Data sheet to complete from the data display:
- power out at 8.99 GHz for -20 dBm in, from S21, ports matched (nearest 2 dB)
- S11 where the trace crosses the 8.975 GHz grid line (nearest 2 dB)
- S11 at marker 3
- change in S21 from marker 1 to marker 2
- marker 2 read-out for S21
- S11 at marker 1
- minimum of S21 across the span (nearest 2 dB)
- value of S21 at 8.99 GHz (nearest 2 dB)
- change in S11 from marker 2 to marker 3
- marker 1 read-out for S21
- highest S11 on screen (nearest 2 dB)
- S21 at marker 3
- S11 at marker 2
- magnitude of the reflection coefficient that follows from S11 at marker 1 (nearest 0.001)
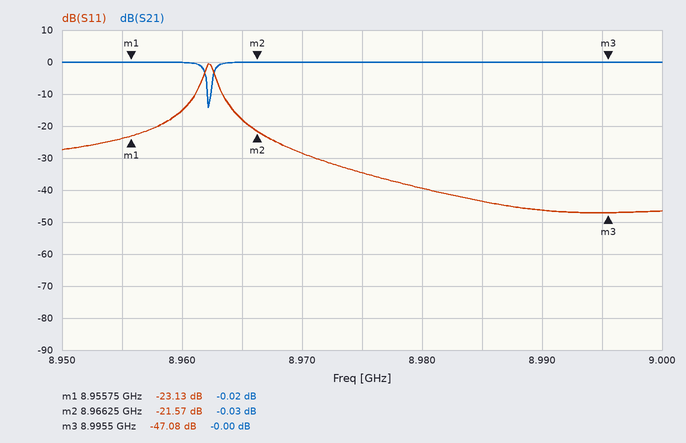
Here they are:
-20 dBm
-34 dB
-47.08 dB
-0.01 dB
-0.03 dB
-23.13 dB
-14 dB
0 dB
-25.51 dB
-0.02 dB
0 dB
-0.00 dB
-21.57 dB
0.070
